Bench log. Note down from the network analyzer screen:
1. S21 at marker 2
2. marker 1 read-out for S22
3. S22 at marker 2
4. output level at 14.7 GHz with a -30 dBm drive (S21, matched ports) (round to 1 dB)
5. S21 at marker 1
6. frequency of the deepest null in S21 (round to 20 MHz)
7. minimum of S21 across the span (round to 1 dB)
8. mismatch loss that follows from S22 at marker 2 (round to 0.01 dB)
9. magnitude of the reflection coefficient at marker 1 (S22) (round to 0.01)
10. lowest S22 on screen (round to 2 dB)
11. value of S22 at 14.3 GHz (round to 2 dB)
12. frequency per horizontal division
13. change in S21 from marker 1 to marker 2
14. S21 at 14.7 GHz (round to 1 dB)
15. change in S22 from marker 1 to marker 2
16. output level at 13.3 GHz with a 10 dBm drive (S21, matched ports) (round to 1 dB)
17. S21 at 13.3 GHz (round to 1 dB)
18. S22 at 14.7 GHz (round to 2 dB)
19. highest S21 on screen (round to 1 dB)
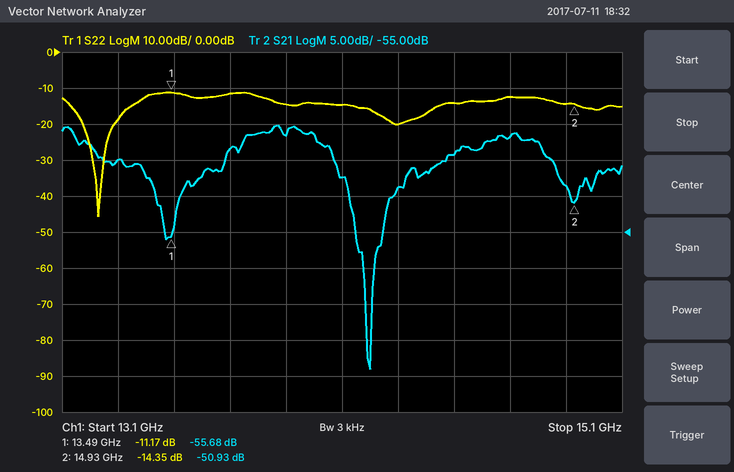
-50.93 dB
-11.17 dB
-14.35 dB
-72 dBm
-55.68 dB
14.20 GHz
-74 dB
0.16 dB
0.28
-46 dB
-20 dB
200 MHz
4.75 dB
-42 dB
-3.18 dB
-35 dBm
-45 dB
-12 dB
-40 dB
